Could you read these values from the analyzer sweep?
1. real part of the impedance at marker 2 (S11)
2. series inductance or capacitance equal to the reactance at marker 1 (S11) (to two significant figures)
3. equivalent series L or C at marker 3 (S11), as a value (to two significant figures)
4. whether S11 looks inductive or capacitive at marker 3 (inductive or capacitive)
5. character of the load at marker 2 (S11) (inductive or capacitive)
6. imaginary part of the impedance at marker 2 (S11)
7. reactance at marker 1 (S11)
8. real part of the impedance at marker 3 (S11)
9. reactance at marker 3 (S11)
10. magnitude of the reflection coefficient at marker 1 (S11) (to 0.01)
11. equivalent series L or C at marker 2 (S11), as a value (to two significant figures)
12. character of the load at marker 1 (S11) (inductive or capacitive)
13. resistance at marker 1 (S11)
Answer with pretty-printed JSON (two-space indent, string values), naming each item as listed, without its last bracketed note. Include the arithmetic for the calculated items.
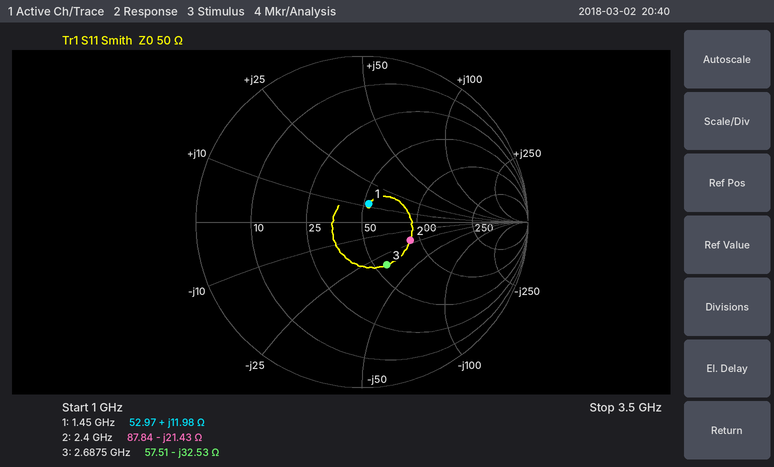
{
  "real part of the impedance at marker 2": "87.84 Ω",
  "series inductance or capacitance equal to the reactance at marker 1 (S11)": "L = 11.98 Ω/(2π × 1.45 GHz) ≈ 1.3 nH",
  "equivalent series L or C at marker 3 (S11), as a value": "C = 1/(2π × 2.6875 GHz × 32.53 Ω) ≈ 1.8 pF",
  "whether S11 looks inductive or capacitive at marker 3": "capacitive",
  "character of the load at marker 2 (S11)": "capacitive",
  "imaginary part of the impedance at marker 2": "-21.43 Ω",
  "reactance at marker 1": "+11.98 Ω",
  "real part of the impedance at marker 3": "57.51 Ω",
  "reactance at marker 3": "-32.53 Ω",
  "magnitude of the reflection coefficient at marker 1 (S11)": "0.12",
  "equivalent series L or C at marker 2 (S11), as a value": "C = 1/(2π × 2.4 GHz × 21.43 Ω) ≈ 3.1 pF",
  "character of the load at marker 1 (S11)": "inductive",
  "resistance at marker 1": "52.97 Ω"
}
